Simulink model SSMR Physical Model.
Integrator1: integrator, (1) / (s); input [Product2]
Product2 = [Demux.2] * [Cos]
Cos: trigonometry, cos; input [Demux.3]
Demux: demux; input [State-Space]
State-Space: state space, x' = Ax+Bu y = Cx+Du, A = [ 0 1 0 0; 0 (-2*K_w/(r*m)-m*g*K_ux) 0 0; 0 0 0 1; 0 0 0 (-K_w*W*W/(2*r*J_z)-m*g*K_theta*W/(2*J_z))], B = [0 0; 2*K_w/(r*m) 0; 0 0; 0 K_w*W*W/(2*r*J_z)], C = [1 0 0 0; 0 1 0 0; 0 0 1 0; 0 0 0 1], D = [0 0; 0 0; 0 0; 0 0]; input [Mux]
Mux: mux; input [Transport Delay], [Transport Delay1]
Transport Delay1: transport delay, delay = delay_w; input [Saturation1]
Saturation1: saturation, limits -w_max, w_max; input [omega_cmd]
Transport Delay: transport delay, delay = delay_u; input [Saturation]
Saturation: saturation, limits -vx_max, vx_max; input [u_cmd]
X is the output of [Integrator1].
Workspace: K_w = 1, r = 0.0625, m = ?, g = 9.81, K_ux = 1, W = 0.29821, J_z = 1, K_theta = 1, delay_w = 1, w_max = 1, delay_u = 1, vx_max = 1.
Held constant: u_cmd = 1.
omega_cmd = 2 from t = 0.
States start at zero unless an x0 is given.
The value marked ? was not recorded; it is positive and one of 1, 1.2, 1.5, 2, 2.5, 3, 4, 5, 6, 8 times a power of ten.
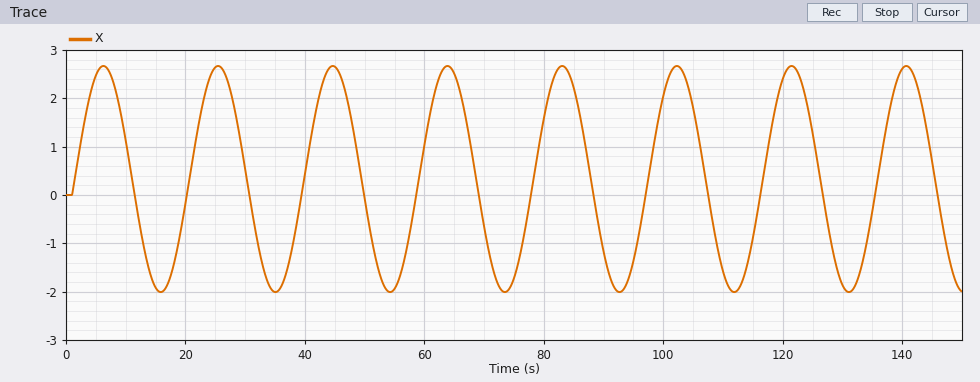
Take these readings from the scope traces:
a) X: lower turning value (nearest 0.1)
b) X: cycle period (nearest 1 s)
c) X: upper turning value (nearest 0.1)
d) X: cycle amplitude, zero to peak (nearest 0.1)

-2.0
19 s
2.7
2.3
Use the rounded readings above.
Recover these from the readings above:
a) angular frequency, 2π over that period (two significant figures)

0.33 rad/s
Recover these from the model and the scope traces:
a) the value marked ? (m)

1
